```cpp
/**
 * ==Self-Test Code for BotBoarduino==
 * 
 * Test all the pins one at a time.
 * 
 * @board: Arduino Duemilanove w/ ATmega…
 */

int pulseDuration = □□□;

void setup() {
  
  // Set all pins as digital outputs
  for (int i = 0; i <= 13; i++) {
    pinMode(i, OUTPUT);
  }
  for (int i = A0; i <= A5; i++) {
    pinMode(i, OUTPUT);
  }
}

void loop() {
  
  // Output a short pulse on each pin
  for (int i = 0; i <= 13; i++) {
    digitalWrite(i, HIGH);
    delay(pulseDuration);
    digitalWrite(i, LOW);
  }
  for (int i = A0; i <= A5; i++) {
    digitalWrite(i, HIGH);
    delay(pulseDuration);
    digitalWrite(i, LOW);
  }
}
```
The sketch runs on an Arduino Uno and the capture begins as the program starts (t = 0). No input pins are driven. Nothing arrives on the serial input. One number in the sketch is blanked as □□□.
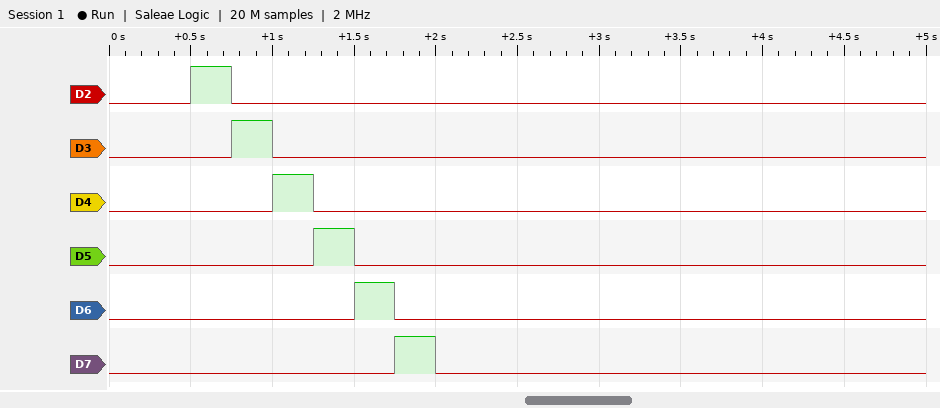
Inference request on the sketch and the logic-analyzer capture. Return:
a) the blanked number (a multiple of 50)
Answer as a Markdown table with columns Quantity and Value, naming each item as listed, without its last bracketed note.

| Quantity | Value |
|---|---|
| the blanked number | 250 |
